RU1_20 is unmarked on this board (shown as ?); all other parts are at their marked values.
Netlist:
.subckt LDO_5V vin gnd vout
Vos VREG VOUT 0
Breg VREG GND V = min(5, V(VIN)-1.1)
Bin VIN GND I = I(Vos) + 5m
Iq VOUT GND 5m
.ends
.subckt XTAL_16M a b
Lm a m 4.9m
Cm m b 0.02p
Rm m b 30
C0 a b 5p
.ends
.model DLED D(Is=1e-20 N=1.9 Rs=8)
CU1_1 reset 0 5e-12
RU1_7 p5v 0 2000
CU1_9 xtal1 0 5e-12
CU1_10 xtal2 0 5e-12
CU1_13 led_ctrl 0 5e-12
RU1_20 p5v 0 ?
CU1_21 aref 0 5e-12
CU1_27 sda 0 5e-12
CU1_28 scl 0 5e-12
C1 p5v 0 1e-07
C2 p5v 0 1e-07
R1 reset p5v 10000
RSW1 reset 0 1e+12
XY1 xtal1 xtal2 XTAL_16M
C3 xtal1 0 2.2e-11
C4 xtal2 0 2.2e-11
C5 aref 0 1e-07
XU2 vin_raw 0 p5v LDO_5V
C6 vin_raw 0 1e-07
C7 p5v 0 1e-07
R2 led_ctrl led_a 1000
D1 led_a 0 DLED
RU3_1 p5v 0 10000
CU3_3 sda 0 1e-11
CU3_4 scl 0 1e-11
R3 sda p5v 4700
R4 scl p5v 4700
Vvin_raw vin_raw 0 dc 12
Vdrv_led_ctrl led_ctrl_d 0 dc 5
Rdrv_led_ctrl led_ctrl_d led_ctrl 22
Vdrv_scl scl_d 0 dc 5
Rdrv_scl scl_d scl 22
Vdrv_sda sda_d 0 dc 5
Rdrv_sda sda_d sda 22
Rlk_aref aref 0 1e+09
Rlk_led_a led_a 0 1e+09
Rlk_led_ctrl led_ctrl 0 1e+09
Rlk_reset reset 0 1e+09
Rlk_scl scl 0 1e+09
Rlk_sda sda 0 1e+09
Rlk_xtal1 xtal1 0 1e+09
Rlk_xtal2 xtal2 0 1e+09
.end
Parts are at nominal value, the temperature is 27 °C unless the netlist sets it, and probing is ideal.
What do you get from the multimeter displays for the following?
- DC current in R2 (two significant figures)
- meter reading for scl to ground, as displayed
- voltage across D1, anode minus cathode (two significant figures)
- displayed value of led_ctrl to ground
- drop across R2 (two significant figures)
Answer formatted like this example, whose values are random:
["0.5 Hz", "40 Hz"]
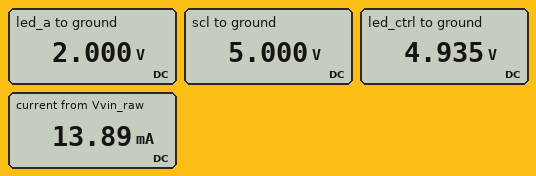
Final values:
["2.9 mA", "5.000 V", "2.0 V", "4.935 V", "2.9 V"]
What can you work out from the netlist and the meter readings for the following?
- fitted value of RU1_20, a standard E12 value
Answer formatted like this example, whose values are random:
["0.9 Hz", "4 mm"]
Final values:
["5.6 kΩ"]
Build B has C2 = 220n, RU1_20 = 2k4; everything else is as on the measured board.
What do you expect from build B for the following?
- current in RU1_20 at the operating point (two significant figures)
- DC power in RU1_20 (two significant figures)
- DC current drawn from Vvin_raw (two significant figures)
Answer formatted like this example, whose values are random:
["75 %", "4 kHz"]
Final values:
["2.1 mA", "10 mW", "15 mA"]
